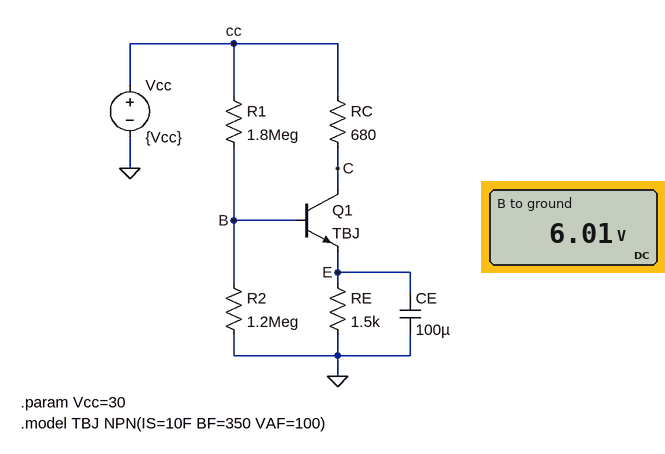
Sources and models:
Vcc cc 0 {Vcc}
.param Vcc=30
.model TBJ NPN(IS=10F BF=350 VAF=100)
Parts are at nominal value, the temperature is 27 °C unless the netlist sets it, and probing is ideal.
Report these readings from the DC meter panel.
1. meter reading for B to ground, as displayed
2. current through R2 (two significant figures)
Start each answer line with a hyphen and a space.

- 6.01 V
- 5.0 µA
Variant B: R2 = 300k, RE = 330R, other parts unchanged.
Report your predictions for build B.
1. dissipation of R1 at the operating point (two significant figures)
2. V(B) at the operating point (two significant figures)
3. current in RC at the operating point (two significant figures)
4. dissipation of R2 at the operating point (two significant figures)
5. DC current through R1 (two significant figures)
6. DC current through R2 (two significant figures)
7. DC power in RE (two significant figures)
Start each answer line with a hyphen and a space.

- 440 µW
- 2.0 V
- 3.9 mA
- 13 µW
- 16 µA
- 6.6 µA
- 5.1 mW
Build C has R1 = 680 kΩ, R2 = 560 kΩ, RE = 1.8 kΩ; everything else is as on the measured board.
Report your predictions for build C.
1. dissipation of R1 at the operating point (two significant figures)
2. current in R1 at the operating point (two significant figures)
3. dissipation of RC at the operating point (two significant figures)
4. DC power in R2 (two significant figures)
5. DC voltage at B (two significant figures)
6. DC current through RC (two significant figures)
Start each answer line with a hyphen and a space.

- 600 µW
- 30 µA
- 17 mW
- 170 µW
- 9.8 V
- 5.0 mA
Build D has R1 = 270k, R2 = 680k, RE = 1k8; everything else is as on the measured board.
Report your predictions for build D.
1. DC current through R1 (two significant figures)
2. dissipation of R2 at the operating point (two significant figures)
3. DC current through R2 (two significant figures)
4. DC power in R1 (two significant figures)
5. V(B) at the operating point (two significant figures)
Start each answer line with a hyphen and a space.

- 49 µA
- 420 µW
- 25 µA
- 640 µW
- 17 V
